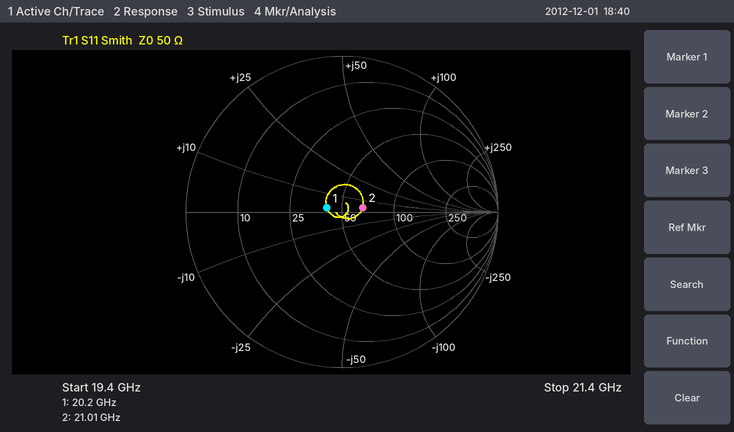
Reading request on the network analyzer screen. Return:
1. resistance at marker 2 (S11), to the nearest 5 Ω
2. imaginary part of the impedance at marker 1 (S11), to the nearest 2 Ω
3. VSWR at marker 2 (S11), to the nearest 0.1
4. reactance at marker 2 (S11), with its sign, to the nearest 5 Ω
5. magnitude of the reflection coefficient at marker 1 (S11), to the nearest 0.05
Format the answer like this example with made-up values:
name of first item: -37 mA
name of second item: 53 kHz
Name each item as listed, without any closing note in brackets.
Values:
resistance at marker 2 (S11), to the nearest 5 Ω: 65 Ω
imaginary part of the impedance at marker 1 (S11), to the nearest 2 Ω: +2 Ω
VSWR at marker 2 (S11), to the nearest 0.1: 1.3
reactance at marker 2 (S11), with its sign, to the nearest 5 Ω: +5 Ω
magnitude of the reflection coefficient at marker 1 (S11), to the nearest 0.05: 0.10
